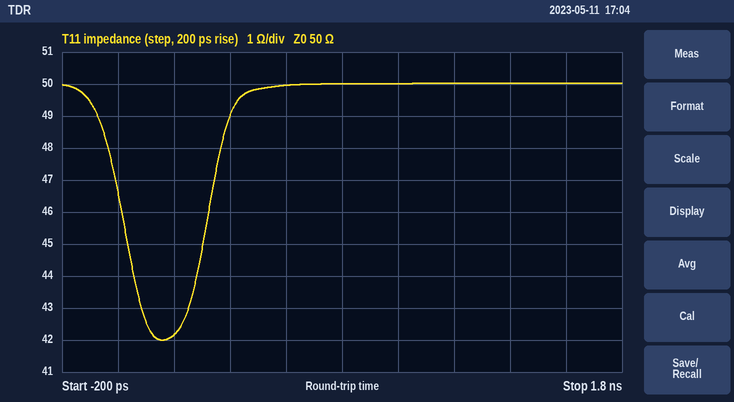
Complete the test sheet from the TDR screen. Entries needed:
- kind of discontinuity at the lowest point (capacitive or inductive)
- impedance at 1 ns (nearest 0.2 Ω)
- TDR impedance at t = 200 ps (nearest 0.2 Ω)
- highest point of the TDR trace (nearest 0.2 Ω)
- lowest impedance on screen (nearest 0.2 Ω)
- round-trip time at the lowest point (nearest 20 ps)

capacitive
50.0 Ω
42.2 Ω
50.0 Ω
42.0 Ω
160 ps
